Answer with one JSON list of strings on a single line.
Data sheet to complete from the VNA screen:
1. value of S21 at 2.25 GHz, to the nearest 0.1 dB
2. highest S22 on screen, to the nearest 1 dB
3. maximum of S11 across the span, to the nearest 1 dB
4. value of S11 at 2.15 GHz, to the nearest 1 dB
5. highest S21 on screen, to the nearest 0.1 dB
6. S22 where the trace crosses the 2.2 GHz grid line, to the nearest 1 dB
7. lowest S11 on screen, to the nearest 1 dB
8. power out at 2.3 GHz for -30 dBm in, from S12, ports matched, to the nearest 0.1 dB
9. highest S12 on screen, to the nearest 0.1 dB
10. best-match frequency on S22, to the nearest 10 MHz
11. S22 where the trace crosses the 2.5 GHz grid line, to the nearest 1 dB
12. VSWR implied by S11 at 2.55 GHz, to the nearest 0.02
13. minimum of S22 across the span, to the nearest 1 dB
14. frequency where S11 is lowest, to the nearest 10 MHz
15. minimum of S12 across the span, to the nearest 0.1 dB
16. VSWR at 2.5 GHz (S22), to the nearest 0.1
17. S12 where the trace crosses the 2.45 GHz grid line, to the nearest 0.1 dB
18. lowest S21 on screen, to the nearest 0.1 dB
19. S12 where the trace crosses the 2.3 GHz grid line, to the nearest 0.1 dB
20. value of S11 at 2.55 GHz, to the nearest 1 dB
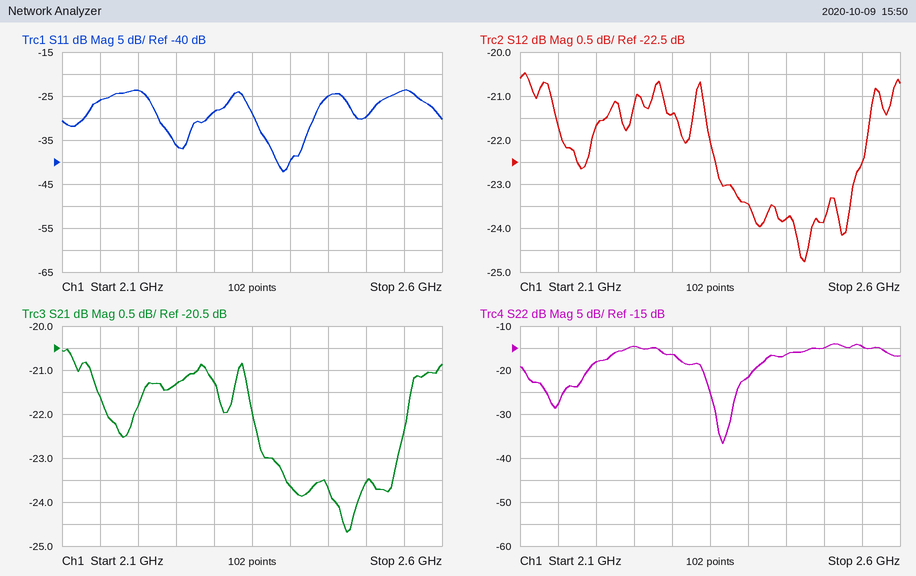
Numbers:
["-21.3 dB", "-14 dB", "-24 dB", "-26 dB", "-20.5 dB", "-18 dB", "-42 dB", "-51.4 dBm", "-20.5 dB", "2.37 GHz", "-15 dB", "1.14", "-37 dB", "2.39 GHz", "-24.8 dB", "1.4", "-23.8 dB", "-24.7 dB", "-21.4 dB", "-24 dB"]
